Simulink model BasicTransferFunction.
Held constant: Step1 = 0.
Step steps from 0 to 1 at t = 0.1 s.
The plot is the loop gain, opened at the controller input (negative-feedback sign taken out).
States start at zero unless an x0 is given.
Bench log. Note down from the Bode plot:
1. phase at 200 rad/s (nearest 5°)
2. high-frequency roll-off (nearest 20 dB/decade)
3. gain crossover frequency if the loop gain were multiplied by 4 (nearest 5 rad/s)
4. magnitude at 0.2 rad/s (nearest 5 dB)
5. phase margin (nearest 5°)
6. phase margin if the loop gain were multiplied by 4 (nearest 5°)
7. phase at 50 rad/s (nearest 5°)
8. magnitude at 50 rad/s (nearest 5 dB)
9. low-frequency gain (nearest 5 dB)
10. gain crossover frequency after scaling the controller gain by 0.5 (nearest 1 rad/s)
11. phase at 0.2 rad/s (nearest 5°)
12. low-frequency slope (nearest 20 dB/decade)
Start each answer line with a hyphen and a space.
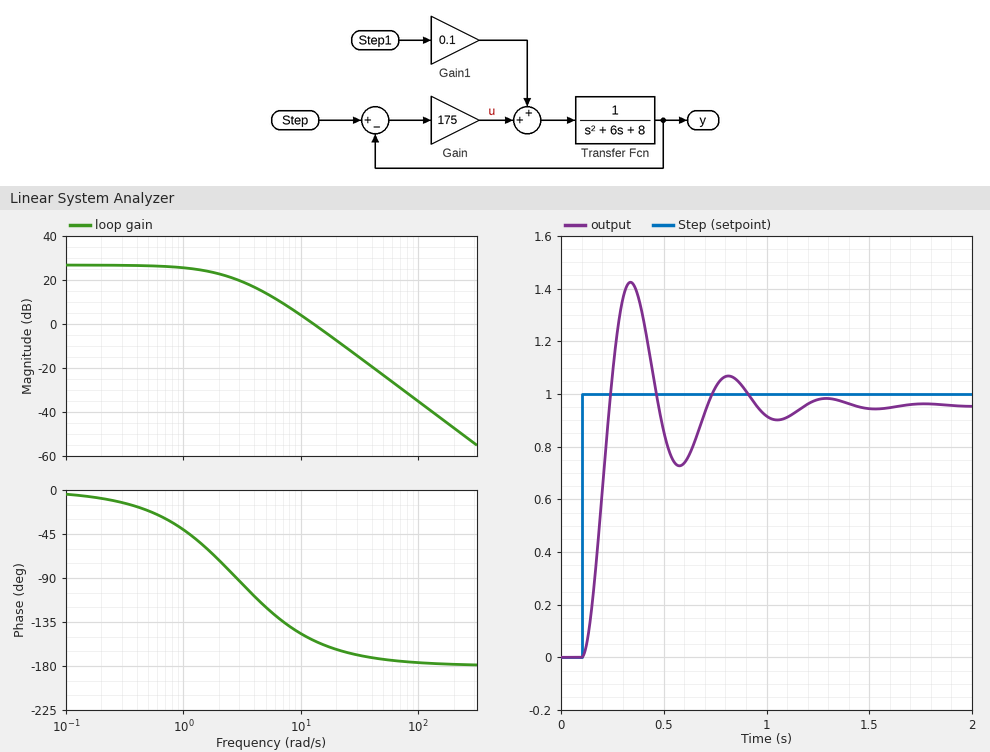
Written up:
- -180°
- -40 dB/decade
- 25 rad/s
- 25 dB
- 25°
- 15°
- -175°
- -25 dB
- 25 dB
- 9 rad/s
- -10°
- 0 dB/decade
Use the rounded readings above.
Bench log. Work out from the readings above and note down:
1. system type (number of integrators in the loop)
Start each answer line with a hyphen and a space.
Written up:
- 0
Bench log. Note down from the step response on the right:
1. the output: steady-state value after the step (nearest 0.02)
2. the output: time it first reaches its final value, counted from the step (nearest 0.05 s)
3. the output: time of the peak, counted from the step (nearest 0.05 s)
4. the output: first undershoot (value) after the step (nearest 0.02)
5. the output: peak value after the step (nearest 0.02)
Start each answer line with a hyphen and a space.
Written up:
- 0.96
- 0.15 s
- 0.25 s
- 0.72
- 1.42
